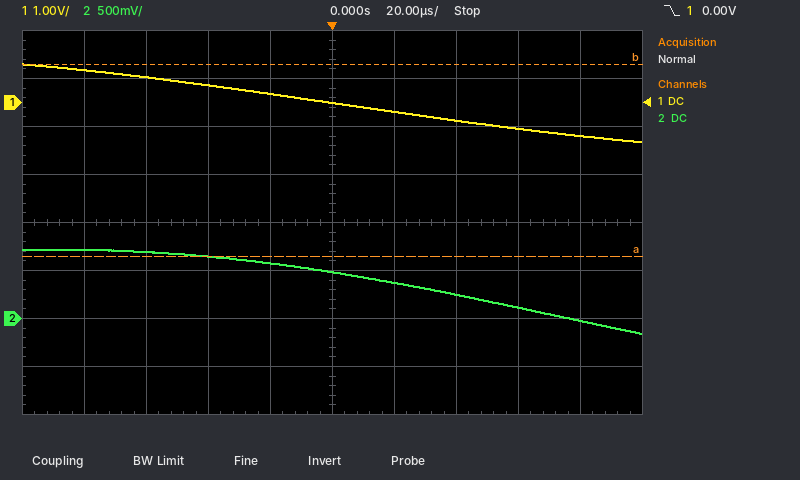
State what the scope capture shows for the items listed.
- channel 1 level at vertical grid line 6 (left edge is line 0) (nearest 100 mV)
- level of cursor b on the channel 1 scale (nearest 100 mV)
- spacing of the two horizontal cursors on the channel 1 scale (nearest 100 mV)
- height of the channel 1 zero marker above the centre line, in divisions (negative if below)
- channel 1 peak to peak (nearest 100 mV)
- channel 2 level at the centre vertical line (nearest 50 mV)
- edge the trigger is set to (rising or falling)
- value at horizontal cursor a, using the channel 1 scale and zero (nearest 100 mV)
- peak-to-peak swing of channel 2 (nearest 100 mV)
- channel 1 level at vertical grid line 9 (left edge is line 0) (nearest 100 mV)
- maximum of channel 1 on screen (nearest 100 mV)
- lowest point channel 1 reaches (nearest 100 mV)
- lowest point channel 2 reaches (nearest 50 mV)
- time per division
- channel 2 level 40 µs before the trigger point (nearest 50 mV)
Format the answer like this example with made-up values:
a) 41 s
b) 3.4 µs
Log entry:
a) -200 mV
b) 800 mV
c) 4.0 V
d) +2.5 div
e) 1.6 V
f) 500 mV
g) falling
h) -3.2 V
i) 900 mV
j) -700 mV
k) 800 mV
l) -800 mV
m) -150 mV
n) 20 µs
o) 650 mV
